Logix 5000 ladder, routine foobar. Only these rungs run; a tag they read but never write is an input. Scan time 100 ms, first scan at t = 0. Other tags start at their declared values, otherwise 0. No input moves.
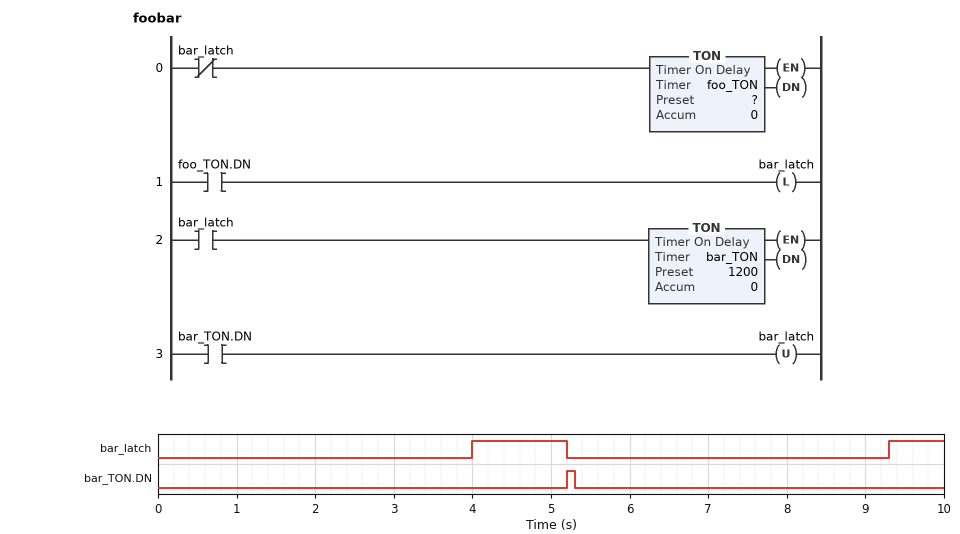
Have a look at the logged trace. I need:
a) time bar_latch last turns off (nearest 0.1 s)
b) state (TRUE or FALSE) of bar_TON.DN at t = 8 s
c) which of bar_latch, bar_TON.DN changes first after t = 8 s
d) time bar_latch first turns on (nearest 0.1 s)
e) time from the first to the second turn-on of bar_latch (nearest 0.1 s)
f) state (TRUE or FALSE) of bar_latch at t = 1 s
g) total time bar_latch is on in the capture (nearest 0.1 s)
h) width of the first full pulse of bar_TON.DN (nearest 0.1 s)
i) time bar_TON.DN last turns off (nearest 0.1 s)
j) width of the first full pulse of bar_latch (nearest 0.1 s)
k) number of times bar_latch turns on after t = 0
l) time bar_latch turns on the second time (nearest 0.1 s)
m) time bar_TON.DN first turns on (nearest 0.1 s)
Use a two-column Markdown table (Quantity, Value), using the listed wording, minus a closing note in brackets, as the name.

| Quantity | Value |
|---|---|
| time bar_latch last turns off | 5.2 s |
| state (TRUE or FALSE) of bar_TON.DN at t = 8 s | FALSE |
| which of bar_latch, bar_TON.DN changes first after t = 8 s | bar_latch |
| time bar_latch first turns on | 4.0 s |
| time from the first to the second turn-on of bar_latch | 5.3 s |
| state (TRUE or FALSE) of bar_latch at t = 1 s | FALSE |
| total time bar_latch is on in the capture | 1.9 s |
| width of the first full pulse of bar_TON.DN | 0.1 s |
| time bar_TON.DN last turns off | 5.3 s |
| width of the first full pulse of bar_latch | 1.2 s |
| number of times bar_latch turns on after t = 0 | 2 |
| time bar_latch turns on the second time | 9.3 s |
| time bar_TON.DN first turns on | 5.2 s |
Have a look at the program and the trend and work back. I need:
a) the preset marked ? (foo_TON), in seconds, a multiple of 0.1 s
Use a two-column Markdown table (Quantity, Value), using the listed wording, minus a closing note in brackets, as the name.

| Quantity | Value |
|---|---|
| the preset marked ? (foo_TON), in seconds, a multiple of 0.1 s | 4.0 s |
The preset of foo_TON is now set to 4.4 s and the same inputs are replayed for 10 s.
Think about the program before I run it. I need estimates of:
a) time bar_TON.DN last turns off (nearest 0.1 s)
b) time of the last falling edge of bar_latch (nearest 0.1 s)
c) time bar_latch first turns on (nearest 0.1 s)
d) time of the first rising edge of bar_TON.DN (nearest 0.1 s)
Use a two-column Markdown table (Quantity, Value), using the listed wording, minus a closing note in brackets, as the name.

| Quantity | Value |
|---|---|
| time bar_TON.DN last turns off | 5.7 s |
| time of the last falling edge of bar_latch | 5.6 s |
| time bar_latch first turns on | 4.4 s |
| time of the first rising edge of bar_TON.DN | 5.6 s |
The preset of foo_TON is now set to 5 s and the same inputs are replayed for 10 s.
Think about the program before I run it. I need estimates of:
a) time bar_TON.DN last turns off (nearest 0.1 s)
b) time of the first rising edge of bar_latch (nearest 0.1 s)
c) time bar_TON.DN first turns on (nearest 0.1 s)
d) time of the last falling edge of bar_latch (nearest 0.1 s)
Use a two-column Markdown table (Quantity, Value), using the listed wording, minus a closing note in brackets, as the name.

| Quantity | Value |
|---|---|
| time bar_TON.DN last turns off | 6.3 s |
| time of the first rising edge of bar_latch | 5.0 s |
| time bar_TON.DN first turns on | 6.2 s |
| time of the last falling edge of bar_latch | 6.2 s |
